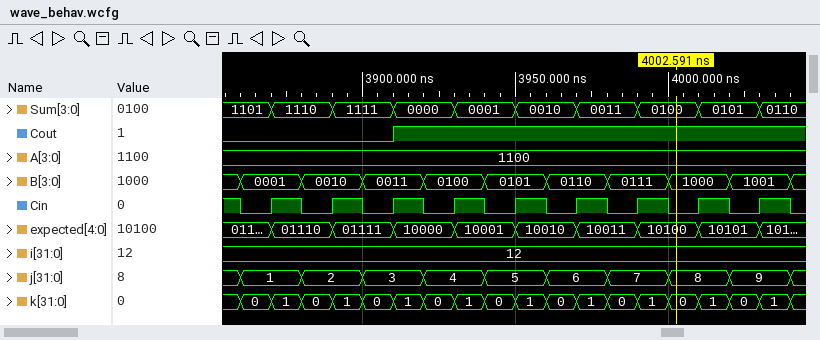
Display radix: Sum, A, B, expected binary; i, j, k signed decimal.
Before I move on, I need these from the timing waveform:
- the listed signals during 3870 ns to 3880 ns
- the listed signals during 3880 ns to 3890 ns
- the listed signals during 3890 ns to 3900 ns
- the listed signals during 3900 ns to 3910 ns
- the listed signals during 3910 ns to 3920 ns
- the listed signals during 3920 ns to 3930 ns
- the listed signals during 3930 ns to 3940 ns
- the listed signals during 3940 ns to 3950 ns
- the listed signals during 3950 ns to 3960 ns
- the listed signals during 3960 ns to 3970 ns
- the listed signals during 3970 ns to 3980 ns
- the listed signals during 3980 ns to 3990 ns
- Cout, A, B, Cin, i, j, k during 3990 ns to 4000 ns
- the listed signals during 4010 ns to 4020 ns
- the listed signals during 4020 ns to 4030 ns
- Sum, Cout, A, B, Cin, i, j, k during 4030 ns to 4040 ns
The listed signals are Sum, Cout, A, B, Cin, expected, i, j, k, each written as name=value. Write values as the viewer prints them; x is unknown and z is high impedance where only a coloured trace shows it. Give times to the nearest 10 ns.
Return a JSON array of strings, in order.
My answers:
["Sum=1110, Cout=0, A=1100, B=0001, Cin=1, expected=01110, i=12, j=1, k=1", "Sum=1110, Cout=0, A=1100, B=0010, Cin=0, expected=01110, i=12, j=2, k=0", "Sum=1111, Cout=0, A=1100, B=0010, Cin=1, expected=01111, i=12, j=2, k=1", "Sum=1111, Cout=0, A=1100, B=0011, Cin=0, expected=01111, i=12, j=3, k=0", "Sum=0000, Cout=1, A=1100, B=0011, Cin=1, expected=10000, i=12, j=3, k=1", "Sum=0000, Cout=1, A=1100, B=0100, Cin=0, expected=10000, i=12, j=4, k=0", "Sum=0001, Cout=1, A=1100, B=0100, Cin=1, expected=10001, i=12, j=4, k=1", "Sum=0001, Cout=1, A=1100, B=0101, Cin=0, expected=10001, i=12, j=5, k=0", "Sum=0010, Cout=1, A=1100, B=0101, Cin=1, expected=10010, i=12, j=5, k=1", "Sum=0010, Cout=1, A=1100, B=0110, Cin=0, expected=10010, i=12, j=6, k=0", "Sum=0011, Cout=1, A=1100, B=0110, Cin=1, expected=10011, i=12, j=6, k=1", "Sum=0011, Cout=1, A=1100, B=0111, Cin=0, expected=10011, i=12, j=7, k=0", "Cout=1, A=1100, B=0111, Cin=1, i=12, j=7, k=1", "Sum=0101, Cout=1, A=1100, B=1000, Cin=1, expected=10101, i=12, j=8, k=1", "Sum=0101, Cout=1, A=1100, B=1001, Cin=0, expected=10101, i=12, j=9, k=0", "Sum=0110, Cout=1, A=1100, B=1001, Cin=1, i=12, j=9, k=1"]
